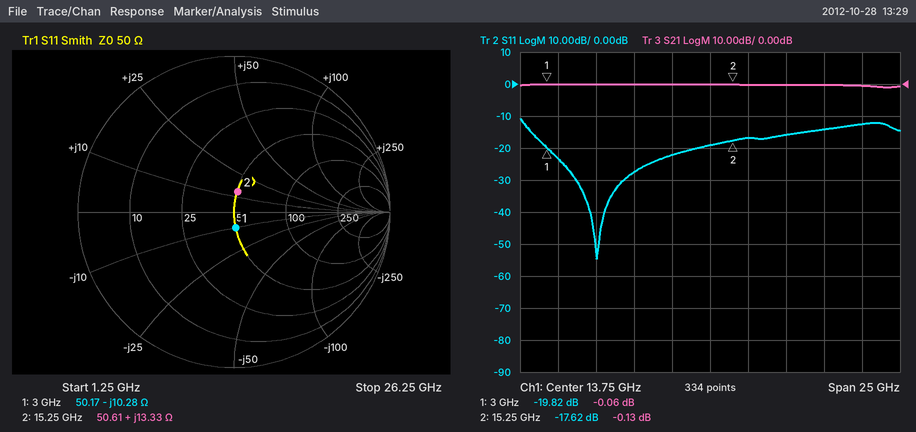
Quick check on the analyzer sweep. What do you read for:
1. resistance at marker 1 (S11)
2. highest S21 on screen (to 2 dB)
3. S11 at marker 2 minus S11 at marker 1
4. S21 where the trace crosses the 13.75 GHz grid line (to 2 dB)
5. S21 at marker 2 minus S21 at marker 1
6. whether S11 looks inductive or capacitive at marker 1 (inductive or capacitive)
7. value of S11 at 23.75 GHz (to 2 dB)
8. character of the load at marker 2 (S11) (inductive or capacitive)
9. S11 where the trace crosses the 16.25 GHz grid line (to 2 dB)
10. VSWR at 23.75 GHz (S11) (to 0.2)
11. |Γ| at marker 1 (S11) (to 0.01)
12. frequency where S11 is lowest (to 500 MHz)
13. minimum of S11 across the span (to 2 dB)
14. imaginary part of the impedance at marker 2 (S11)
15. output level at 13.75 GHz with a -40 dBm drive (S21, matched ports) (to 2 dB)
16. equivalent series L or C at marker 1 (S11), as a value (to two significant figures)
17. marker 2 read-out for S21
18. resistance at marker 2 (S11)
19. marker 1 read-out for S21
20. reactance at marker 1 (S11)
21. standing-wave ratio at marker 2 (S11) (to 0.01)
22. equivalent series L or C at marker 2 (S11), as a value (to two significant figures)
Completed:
50.17 Ω
0 dB
2.20 dB
0 dB
-0.07 dB
capacitive
-12 dB
inductive
-16 dB
1.6
0.10
6.5 GHz
-54 dB
+13.33 Ω
-40 dBm
5.2 pF
-0.13 dB
50.61 Ω
-0.06 dB
-10.28 Ω
1.30
140 pH
